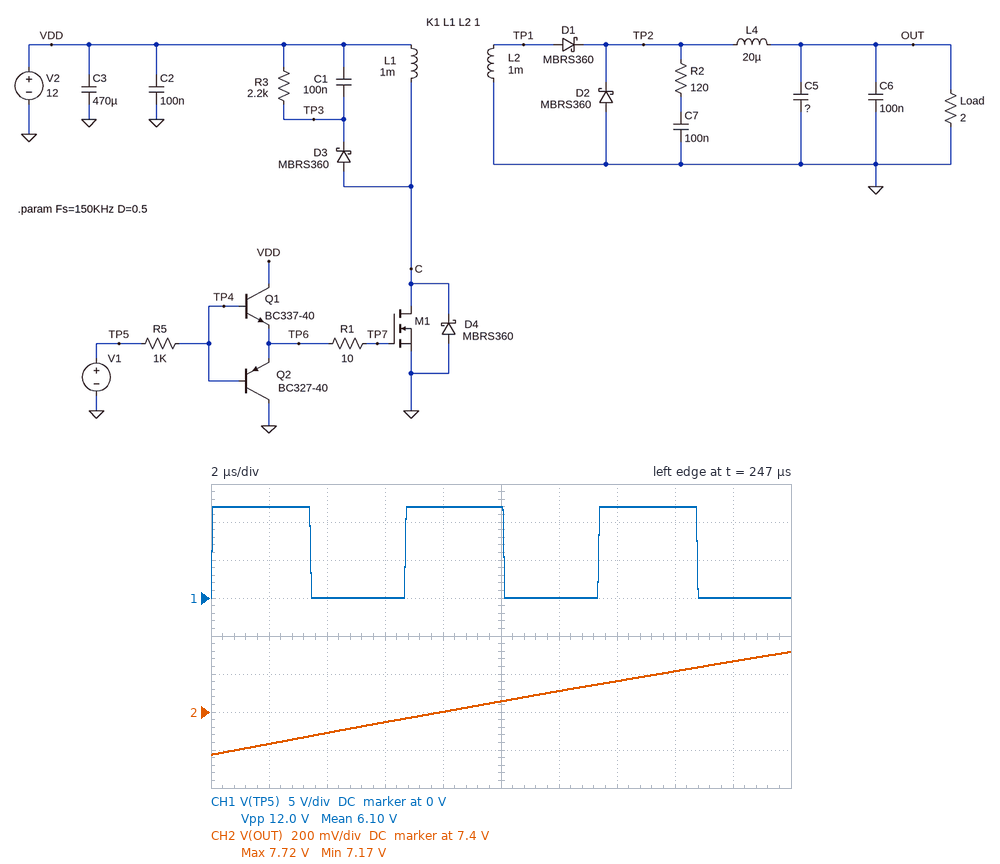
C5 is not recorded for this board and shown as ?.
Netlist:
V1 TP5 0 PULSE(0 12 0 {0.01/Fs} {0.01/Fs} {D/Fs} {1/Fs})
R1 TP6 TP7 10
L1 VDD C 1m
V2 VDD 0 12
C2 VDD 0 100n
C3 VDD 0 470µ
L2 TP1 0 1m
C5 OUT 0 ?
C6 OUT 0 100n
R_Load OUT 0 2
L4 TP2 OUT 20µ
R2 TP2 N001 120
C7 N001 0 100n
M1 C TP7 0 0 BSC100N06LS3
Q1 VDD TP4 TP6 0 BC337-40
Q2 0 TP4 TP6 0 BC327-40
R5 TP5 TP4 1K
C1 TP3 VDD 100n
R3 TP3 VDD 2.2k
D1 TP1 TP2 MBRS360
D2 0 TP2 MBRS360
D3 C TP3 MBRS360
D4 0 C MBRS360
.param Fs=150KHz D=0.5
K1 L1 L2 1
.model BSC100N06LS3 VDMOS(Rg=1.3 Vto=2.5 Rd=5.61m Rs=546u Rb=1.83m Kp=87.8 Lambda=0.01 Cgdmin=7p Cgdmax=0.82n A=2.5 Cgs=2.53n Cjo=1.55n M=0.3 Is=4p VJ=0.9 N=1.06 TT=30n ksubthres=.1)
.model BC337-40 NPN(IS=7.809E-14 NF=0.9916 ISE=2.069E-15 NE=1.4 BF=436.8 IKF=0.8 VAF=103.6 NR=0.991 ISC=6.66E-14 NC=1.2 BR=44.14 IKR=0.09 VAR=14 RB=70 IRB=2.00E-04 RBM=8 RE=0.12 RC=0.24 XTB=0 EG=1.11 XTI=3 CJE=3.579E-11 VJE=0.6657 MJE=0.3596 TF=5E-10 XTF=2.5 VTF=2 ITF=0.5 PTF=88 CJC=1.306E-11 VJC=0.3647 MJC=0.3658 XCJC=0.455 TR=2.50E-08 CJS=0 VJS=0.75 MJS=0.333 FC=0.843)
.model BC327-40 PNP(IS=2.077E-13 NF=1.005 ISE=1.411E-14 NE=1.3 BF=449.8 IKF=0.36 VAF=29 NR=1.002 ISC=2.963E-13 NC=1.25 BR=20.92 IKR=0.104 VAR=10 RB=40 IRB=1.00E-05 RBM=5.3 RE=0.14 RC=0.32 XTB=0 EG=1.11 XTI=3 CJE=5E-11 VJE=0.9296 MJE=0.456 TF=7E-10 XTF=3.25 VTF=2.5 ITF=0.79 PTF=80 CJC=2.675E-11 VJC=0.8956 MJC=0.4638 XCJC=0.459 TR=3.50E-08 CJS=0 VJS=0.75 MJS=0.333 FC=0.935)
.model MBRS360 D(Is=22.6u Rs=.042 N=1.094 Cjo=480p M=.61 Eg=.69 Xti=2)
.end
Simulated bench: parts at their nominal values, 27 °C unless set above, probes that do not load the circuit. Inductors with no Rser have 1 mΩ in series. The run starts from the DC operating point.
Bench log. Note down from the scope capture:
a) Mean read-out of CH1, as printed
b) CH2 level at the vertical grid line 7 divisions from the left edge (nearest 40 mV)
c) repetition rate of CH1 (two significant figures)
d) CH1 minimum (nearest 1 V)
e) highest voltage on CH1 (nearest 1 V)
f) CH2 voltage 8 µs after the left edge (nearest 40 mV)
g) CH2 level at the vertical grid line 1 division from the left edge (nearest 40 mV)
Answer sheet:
6.10 V
7.56 V
150 kHz
0 V
12 V
7.40 V
7.24 V
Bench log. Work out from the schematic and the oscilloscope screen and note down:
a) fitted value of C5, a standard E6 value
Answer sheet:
680 µF
